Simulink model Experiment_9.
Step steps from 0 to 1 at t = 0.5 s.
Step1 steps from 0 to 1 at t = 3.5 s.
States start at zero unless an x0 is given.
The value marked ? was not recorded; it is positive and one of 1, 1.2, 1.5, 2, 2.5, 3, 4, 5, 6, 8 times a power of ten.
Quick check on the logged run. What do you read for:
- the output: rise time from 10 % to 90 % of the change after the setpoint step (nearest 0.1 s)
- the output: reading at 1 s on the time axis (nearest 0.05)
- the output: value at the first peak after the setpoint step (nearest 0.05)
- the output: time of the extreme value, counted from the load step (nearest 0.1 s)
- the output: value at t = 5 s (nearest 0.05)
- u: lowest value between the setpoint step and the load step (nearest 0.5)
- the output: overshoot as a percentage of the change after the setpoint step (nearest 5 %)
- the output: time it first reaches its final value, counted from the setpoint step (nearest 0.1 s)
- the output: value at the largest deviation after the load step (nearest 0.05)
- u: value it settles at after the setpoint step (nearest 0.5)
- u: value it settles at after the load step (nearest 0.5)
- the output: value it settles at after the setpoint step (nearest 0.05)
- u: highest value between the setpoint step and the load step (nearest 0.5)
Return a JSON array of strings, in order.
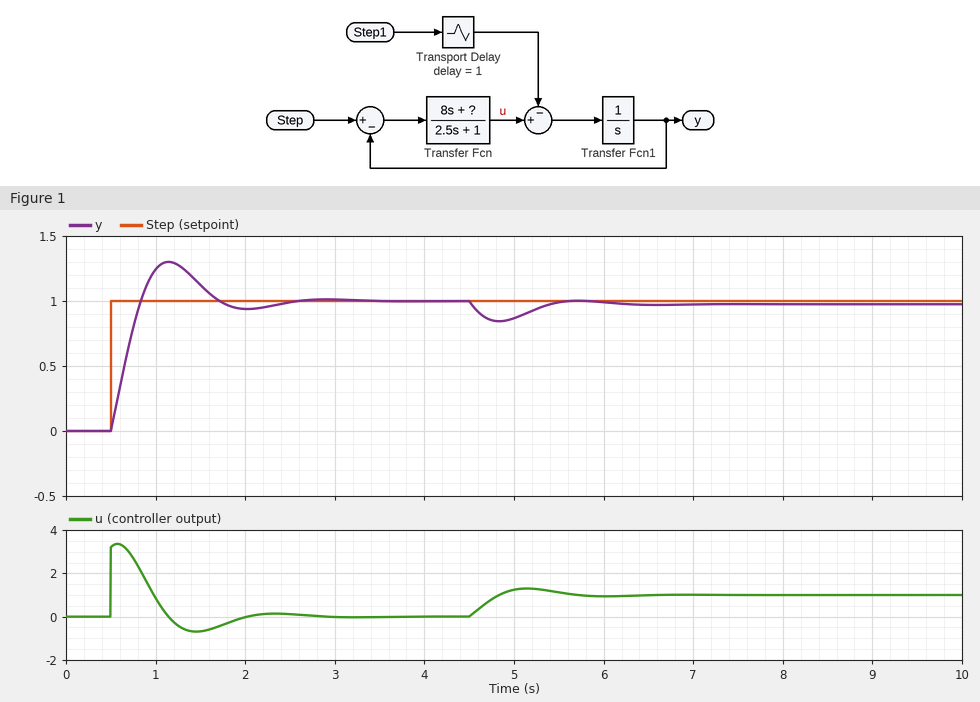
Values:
["0.3 s", "1.25", "1.30", "1.3 s", "0.85", "-0.5", "30 %", "0.3 s", "0.85", "0.0", "1.0", "1.00", "3.5"]
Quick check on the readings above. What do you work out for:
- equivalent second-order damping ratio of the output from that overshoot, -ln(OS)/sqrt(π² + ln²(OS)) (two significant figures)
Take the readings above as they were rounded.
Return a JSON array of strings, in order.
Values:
["0.36"]
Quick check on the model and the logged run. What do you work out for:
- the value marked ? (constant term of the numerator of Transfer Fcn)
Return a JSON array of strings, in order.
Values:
["40"]
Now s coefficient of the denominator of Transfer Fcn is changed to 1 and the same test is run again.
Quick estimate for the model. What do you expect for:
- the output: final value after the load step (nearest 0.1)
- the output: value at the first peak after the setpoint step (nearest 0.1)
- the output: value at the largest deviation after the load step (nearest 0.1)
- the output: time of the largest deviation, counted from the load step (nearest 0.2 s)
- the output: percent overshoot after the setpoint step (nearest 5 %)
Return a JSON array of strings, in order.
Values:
["1.0", "1.2", "0.9", "1.2 s", "15 %"]
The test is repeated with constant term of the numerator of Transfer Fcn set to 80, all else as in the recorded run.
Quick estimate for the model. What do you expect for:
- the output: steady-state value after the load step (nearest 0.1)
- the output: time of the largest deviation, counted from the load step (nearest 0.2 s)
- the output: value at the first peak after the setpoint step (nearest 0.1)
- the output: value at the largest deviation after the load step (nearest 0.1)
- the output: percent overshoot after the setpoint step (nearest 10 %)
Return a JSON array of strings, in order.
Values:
["1.0", "1.2 s", "1.4", "0.9", "40 %"]
